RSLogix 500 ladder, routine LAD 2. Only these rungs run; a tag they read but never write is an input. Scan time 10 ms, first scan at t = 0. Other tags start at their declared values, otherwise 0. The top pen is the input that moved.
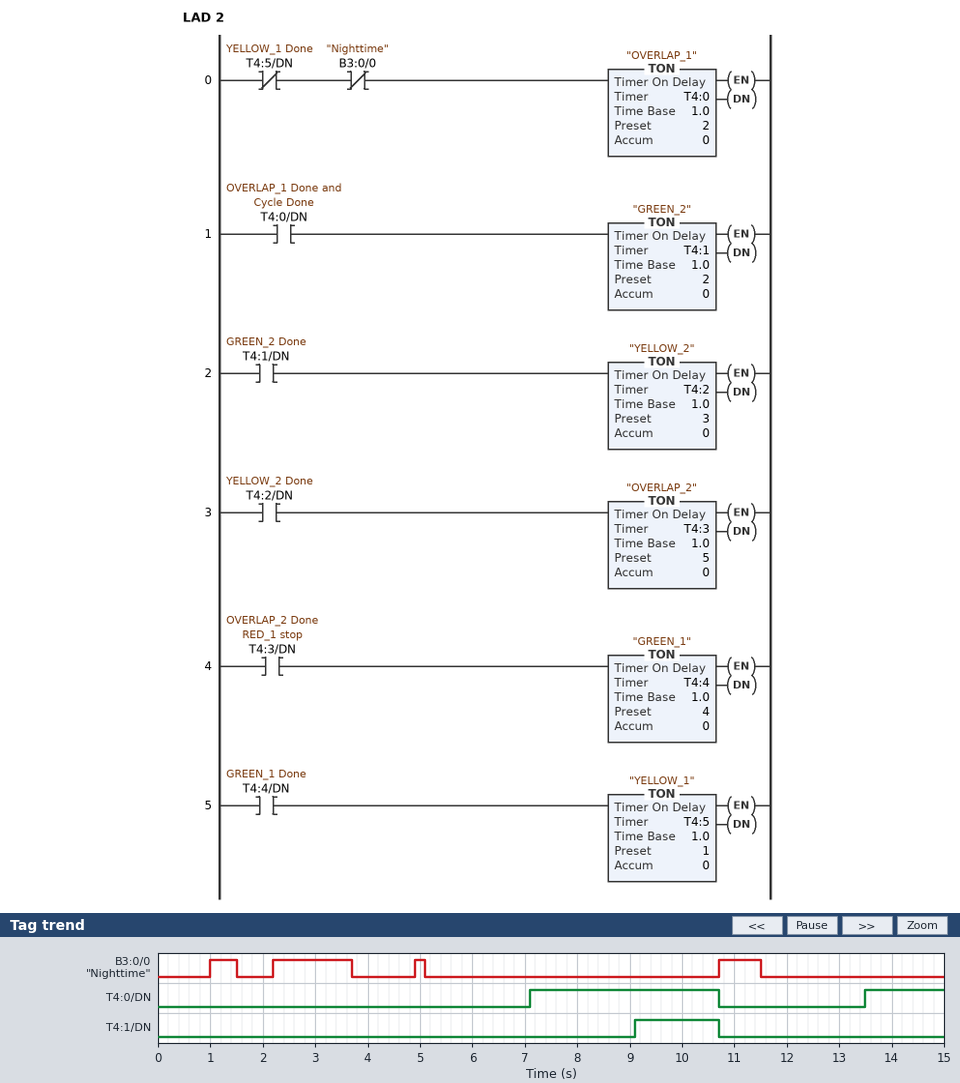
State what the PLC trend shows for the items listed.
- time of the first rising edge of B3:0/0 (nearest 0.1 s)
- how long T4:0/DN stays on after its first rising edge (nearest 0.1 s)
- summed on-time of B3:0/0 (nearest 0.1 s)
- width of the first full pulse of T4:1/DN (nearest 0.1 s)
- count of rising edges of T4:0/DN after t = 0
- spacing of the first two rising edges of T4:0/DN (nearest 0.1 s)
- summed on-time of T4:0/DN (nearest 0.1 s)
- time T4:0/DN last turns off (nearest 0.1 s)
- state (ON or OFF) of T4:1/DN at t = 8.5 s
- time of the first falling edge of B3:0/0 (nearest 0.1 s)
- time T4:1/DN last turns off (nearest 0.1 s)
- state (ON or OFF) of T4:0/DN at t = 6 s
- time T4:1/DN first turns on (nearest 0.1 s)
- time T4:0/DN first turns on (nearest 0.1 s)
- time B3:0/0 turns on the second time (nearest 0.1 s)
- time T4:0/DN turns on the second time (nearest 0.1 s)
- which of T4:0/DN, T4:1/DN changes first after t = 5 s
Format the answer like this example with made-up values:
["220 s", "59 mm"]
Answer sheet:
["1.0 s", "3.6 s", "3.0 s", "1.6 s", "2", "6.4 s", "5.1 s", "10.7 s", "OFF", "1.5 s", "10.7 s", "OFF", "9.1 s", "7.1 s", "2.2 s", "13.5 s", "T4:0/DN"]
